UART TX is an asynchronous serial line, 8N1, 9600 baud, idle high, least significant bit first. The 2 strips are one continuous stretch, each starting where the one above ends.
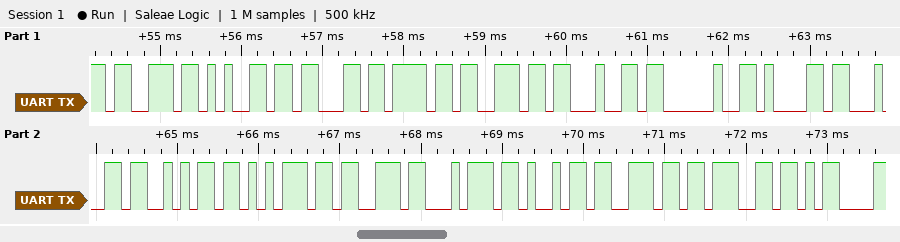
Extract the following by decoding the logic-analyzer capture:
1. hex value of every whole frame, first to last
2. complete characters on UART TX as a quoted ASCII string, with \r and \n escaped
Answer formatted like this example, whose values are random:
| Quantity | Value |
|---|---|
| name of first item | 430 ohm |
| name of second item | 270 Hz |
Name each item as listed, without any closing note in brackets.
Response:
| Quantity | Value |
|---|---|
| hex value of every whole frame, first to last | 0x73 0x65 0x63 0x6F 0x6E 0x64 0x20 0x61 0x64 0x6A 0x75 0x73 0x74 0x69 0x6E 0x67 0x0D |
| complete characters on UART TX as a quoted ASCII string, with \r and \n escaped | "second adjusting\r" |
